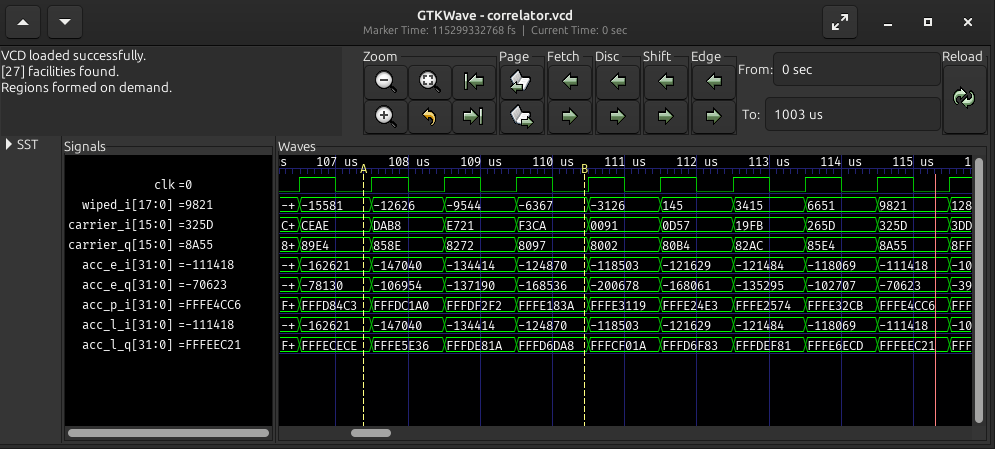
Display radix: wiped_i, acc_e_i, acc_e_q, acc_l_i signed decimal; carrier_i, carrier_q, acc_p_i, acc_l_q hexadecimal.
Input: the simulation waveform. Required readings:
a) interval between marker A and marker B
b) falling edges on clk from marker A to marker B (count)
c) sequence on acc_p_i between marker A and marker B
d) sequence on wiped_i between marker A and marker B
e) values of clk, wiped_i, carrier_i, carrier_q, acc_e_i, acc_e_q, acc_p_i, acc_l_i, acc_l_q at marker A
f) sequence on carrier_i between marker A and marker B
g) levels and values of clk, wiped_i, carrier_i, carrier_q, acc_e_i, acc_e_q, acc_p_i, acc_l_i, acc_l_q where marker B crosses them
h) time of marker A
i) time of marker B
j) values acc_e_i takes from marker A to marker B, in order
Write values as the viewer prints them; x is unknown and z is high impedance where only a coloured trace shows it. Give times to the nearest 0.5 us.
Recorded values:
3 us
3
FFFD84C3, FFFDC1A0, FFFDF2F2, FFFE183A
-15581, -12626, -9544, -6367
clk=0, wiped_i=-15581, carrier_i=CEAE, carrier_q=89E4, acc_e_i=-162621, acc_e_q=-78130, acc_p_i=FFFD84C3, acc_l_i=-162621, acc_l_q=FFFECECE
CEAE, DAB8, E721, F3CA
clk=0, wiped_i=-6367, carrier_i=F3CA, carrier_q=8097, acc_e_i=-124870, acc_e_q=-168536, acc_p_i=FFFE183A, acc_l_i=-124870, acc_l_q=FFFD6DA8
107.5 us
110.5 us
-162621, -147040, -134414, -124870
